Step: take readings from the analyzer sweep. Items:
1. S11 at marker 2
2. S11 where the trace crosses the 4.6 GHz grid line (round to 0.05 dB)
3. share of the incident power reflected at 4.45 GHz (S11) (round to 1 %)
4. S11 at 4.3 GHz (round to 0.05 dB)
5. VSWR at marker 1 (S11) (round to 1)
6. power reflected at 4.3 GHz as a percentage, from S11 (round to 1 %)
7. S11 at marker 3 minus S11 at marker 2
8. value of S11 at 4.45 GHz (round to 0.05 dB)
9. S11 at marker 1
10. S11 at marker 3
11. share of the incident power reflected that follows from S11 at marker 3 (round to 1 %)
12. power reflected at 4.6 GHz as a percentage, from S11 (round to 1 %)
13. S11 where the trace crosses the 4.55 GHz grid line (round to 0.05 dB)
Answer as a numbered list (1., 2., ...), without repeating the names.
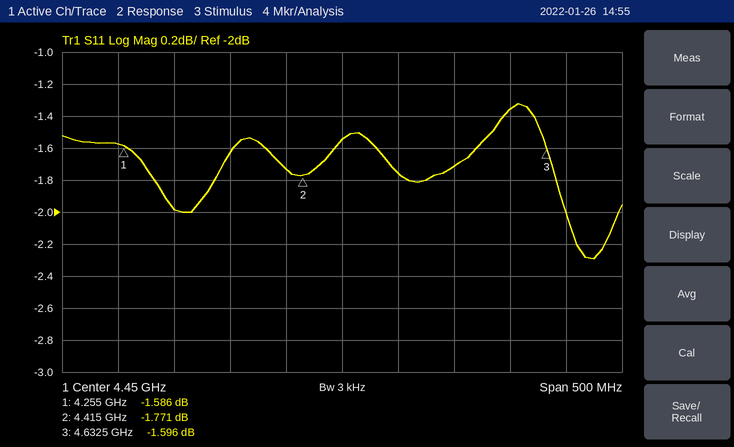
1. -1.771 dB
2. -1.35 dB
3. 70 %
4. -2.00 dB
5. 11
6. 63 %
7. 0.175 dB
8. -1.55 dB
9. -1.586 dB
10. -1.596 dB
11. 69 %
12. 73 %
13. -1.70 dB
